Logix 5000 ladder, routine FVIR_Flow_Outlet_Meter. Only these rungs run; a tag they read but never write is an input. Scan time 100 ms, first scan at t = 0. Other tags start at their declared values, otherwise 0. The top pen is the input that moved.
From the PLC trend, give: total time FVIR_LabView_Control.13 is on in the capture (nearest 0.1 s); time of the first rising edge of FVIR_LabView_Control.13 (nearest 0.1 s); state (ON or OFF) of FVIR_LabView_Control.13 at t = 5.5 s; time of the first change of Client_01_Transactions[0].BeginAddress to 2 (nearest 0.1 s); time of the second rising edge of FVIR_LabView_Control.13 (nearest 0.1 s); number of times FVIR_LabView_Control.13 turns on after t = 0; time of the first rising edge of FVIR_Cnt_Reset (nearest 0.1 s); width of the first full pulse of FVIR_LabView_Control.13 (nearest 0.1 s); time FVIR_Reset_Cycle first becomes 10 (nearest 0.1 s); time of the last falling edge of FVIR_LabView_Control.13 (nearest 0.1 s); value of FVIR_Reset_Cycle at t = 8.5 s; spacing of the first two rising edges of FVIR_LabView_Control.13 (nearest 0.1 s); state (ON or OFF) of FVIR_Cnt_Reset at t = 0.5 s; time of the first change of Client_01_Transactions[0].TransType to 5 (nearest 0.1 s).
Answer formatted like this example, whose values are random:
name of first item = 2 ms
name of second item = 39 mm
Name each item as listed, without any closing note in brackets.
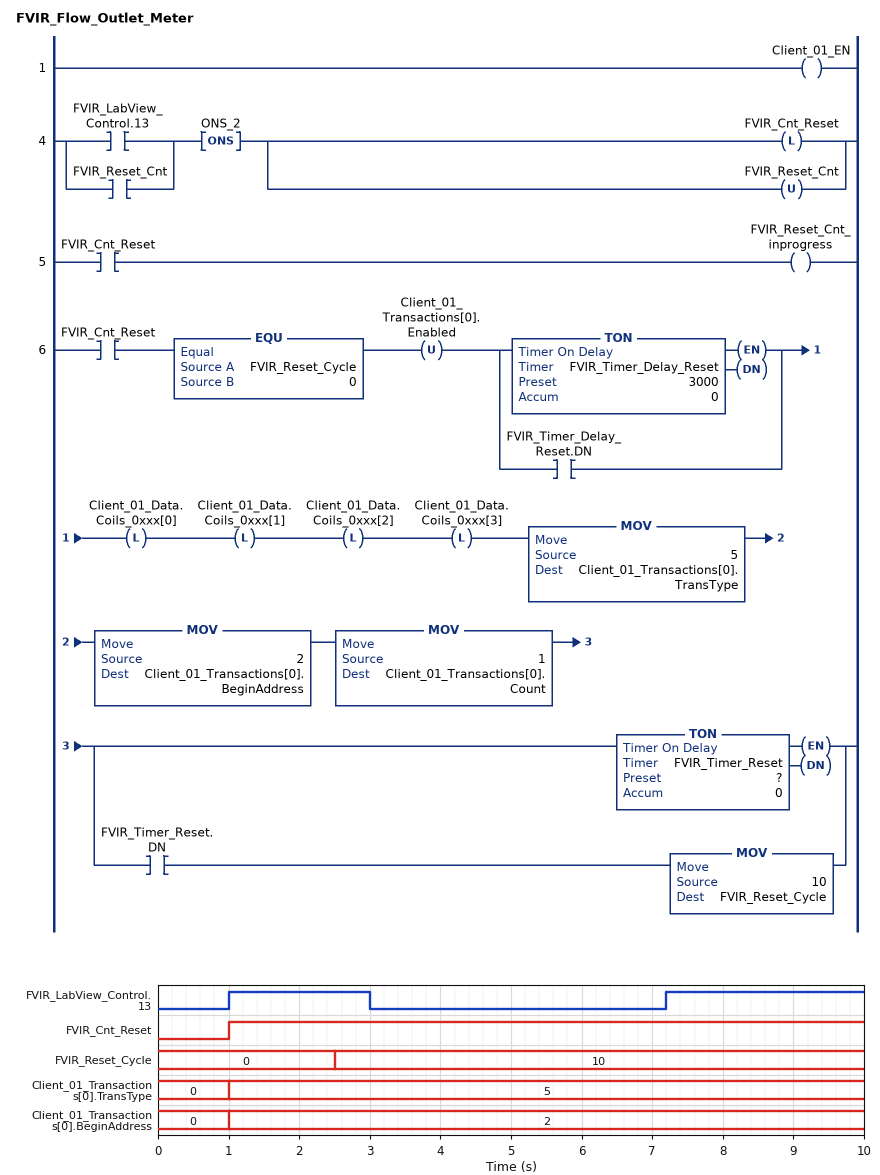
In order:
total time FVIR_LabView_Control.13 is on in the capture = 4.8 s
time of the first rising edge of FVIR_LabView_Control.13 = 1.0 s
state (ON or OFF) of FVIR_LabView_Control.13 at t = 5.5 s = OFF
time of the first change of Client_01_Transactions[0].BeginAddress to 2 = 1.0 s
time of the second rising edge of FVIR_LabView_Control.13 = 7.2 s
number of times FVIR_LabView_Control.13 turns on after t = 0 = 2
time of the first rising edge of FVIR_Cnt_Reset = 1.0 s
width of the first full pulse of FVIR_LabView_Control.13 = 2.0 s
time FVIR_Reset_Cycle first becomes 10 = 2.5 s
time of the last falling edge of FVIR_LabView_Control.13 = 3.0 s
value of FVIR_Reset_Cycle at t = 8.5 s = 10
spacing of the first two rising edges of FVIR_LabView_Control.13 = 6.2 s
state (ON or OFF) of FVIR_Cnt_Reset at t = 0.5 s = OFF
time of the first change of Client_01_Transactions[0].TransType to 5 = 1.0 s
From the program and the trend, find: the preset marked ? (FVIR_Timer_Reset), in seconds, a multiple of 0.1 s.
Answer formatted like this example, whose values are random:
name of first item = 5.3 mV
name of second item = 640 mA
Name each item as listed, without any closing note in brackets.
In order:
the preset marked ? (FVIR_Timer_Reset), in seconds, a multiple of 0.1 s = 1.5 s
